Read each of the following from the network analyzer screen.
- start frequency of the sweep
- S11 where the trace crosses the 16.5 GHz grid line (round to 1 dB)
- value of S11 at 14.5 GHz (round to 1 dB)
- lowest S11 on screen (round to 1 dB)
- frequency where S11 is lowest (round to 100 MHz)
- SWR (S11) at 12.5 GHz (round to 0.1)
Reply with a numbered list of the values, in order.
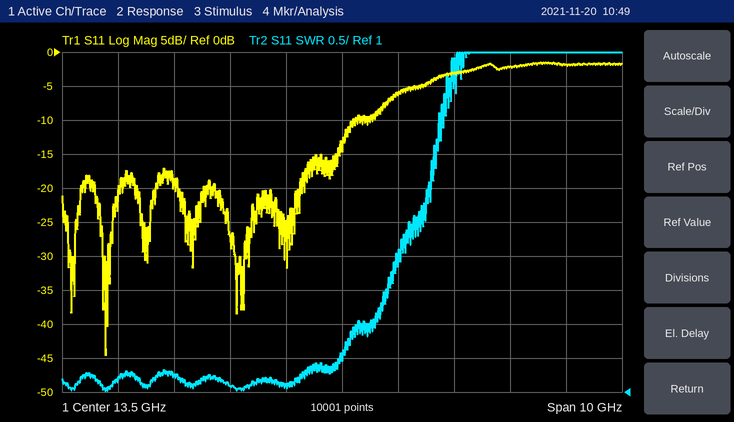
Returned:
1. 8.5 GHz
2. -2 dB
3. -6 dB
4. -45 dB
5. 9.3 GHz
6. 1.1
